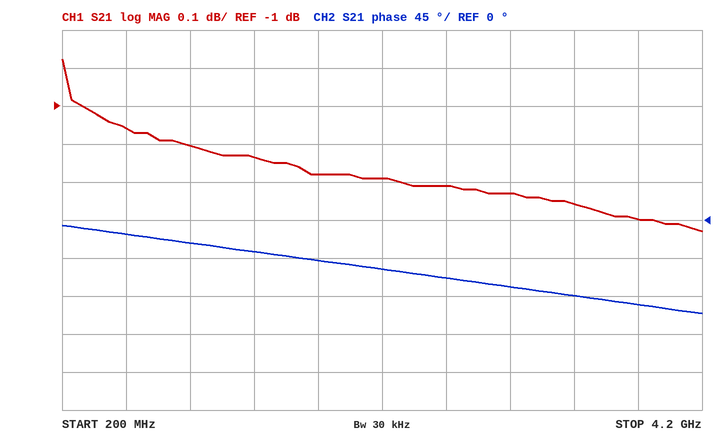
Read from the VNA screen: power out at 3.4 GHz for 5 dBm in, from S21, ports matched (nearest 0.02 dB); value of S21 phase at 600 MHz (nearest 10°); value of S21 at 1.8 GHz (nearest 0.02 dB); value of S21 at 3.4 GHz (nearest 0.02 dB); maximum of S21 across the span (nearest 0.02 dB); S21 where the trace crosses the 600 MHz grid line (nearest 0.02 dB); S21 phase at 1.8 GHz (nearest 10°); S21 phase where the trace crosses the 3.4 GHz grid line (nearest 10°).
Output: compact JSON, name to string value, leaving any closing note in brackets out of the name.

{"power out at 3.4 GHz for 5 dBm in, from S21, ports matched": "3.74 dBm", "value of S21 phase at 600 MHz": "-20°", "value of S21 at 1.8 GHz": "-1.18 dB", "value of S21 at 3.4 GHz": "-1.26 dB", "maximum of S21 across the span": "-0.88 dB", "S21 where the trace crosses the 600 MHz grid line": "-1.06 dB", "S21 phase at 1.8 GHz": "-50°", "S21 phase where the trace crosses the 3.4 GHz grid line": "-90°"}
